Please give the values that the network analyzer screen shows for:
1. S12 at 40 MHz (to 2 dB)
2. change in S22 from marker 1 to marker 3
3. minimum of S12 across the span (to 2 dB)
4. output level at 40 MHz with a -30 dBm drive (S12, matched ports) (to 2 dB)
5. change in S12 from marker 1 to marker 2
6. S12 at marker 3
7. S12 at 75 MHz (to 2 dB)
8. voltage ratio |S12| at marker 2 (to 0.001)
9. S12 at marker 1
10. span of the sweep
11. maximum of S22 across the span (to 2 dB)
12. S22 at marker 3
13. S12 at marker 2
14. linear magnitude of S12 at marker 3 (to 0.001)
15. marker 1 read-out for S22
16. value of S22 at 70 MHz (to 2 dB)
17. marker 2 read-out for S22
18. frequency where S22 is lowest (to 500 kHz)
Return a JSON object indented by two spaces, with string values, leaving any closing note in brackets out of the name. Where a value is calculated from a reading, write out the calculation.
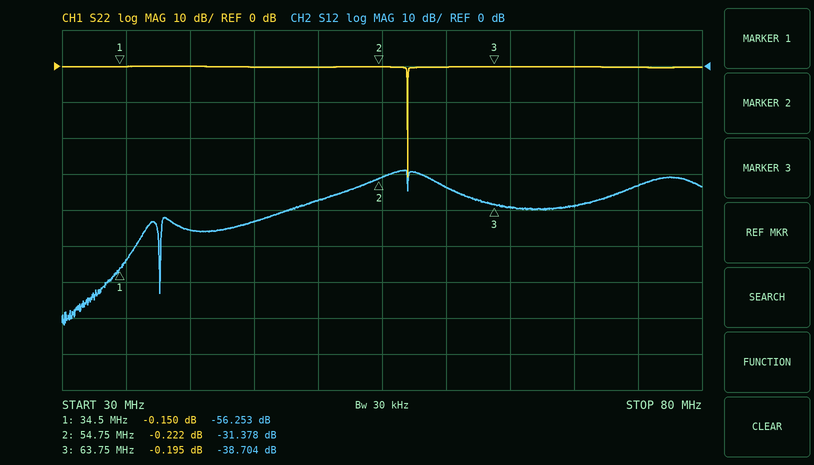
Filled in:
{
  "S12 at 40 MHz": "-46 dB",
  "change in S22 from marker 1 to marker 3": "-0.195 − (-0.15) = -0.045 dB",
  "minimum of S12 across the span": "-72 dB",
  "output level at 40 MHz with a -30 dBm drive (S12, matched ports)": "-30 dBm + (-46 dB) = -76 dBm",
  "change in S12 from marker 1 to marker 2": "-31.378 − (-56.253) = 24.875 dB",
  "S12 at marker 3": "-38.704 dB",
  "S12 at 75 MHz": "-34 dB",
  "voltage ratio |S12| at marker 2": "10^(-31.378/20) ≈ 0.027",
  "S12 at marker 1": "-56.253 dB",
  "span of the sweep": "50 MHz",
  "maximum of S22 across the span": "0 dB",
  "S22 at marker 3": "-0.195 dB",
  "S12 at marker 2": "-31.378 dB",
  "linear magnitude of S12 at marker 3": "10^(-38.704/20) ≈ 0.012",
  "marker 1 read-out for S22": "-0.150 dB",
  "value of S22 at 70 MHz": "0 dB",
  "marker 2 read-out for S22": "-0.222 dB",
  "frequency where S22 is lowest": "57.0 MHz"
}
